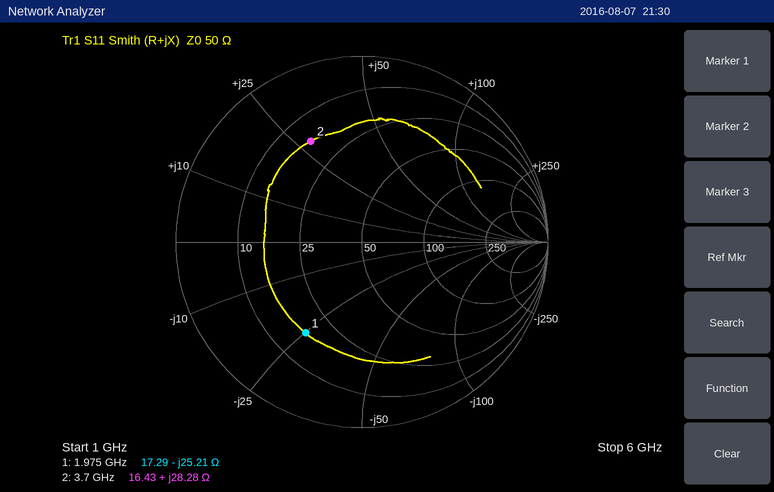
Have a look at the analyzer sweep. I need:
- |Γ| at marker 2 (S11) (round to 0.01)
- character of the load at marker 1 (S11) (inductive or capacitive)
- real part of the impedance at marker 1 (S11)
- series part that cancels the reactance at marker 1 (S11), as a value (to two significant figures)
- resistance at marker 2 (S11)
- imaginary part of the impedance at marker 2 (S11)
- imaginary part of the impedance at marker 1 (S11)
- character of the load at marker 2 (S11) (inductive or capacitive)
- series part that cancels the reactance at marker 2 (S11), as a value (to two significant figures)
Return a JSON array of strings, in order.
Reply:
["0.61", "capacitive", "17.29 Ω", "2.0 nH", "16.43 Ω", "+28.28 Ω", "-25.21 Ω", "inductive", "1.5 pF"]
